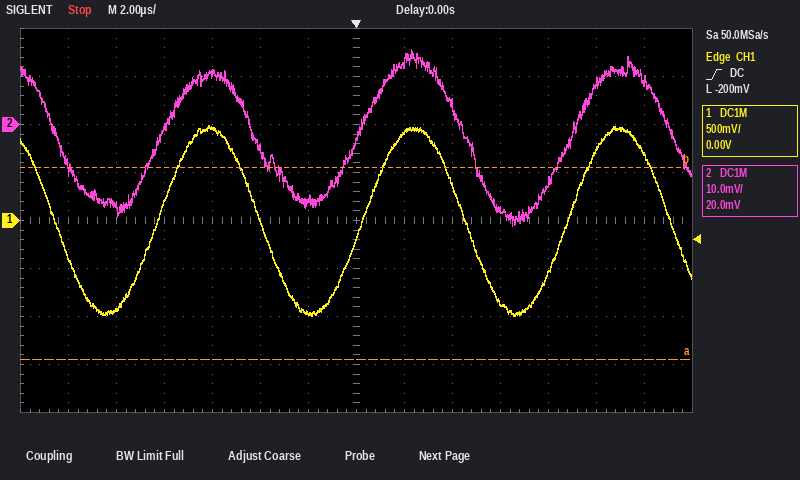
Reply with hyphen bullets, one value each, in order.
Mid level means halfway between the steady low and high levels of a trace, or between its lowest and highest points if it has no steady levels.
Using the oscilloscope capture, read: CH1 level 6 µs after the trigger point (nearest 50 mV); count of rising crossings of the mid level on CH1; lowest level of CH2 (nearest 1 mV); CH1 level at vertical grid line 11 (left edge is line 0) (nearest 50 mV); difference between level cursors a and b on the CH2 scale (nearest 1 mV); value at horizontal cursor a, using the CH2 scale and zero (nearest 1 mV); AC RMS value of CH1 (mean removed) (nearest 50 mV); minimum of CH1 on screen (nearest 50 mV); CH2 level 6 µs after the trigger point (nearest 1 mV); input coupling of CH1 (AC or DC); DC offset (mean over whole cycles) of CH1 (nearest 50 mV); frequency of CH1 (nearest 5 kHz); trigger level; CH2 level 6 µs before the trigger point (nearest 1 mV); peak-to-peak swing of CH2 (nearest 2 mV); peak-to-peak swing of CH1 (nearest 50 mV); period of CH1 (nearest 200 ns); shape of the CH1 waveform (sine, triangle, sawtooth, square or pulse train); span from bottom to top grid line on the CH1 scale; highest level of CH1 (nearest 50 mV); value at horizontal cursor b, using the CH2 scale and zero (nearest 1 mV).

- -850 mV
- 3
- -21 mV
- -550 mV
- 40 mV
- -49 mV
- 700 mV
- -1.00 V
- -18 mV
- DC
- 0 mV
- 115 kHz
- -200 mV
- 11 mV
- 36 mV
- 2.00 V
- 8.6 µs
- sine
- 4 V
- 1.00 V
- -9 mV
